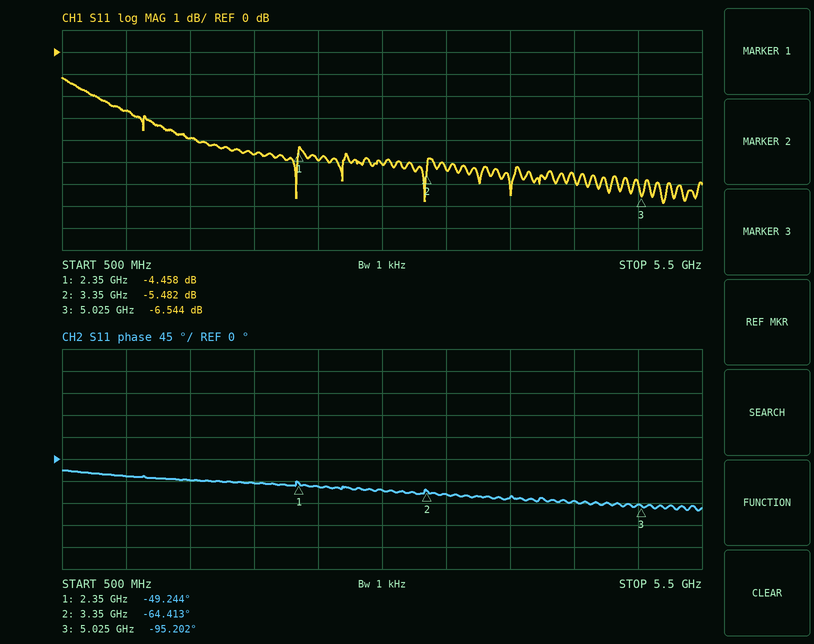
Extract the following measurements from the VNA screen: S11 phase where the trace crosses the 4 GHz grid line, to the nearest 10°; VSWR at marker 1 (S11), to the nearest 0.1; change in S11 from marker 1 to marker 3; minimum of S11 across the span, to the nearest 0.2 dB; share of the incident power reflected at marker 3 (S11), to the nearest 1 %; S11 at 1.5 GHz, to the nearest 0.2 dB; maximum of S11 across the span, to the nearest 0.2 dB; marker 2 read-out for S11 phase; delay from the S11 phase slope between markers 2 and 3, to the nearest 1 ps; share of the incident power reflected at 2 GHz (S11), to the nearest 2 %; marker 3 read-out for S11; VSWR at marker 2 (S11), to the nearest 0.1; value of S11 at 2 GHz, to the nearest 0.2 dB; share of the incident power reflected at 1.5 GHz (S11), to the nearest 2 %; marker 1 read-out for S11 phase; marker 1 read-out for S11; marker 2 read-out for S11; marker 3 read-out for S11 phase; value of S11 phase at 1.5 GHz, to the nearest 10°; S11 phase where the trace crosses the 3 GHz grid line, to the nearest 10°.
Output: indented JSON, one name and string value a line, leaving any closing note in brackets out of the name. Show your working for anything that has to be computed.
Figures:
{
  "S11 phase where the trace crosses the 4 GHz grid line, to the nearest 10°": "-80°",
  "VSWR at marker 1 (S11), to the nearest 0.1": "(1 + 0.5985)/(1 − 0.5985) ≈ 4.0",
  "change in S11 from marker 1 to marker 3": "-6.544 − (-4.458) = -2.086 dB",
  "minimum of S11 across the span, to the nearest 0.2 dB": "-6.8 dB",
  "share of the incident power reflected at marker 3 (S11), to the nearest 1 %": "10^(-6.544/10) ≈ 22 %",
  "S11 at 1.5 GHz, to the nearest 0.2 dB": "-4.0 dB",
  "maximum of S11 across the span, to the nearest 0.2 dB": "-1.2 dB",
  "marker 2 read-out for S11 phase": "-64.413°",
  "delay from the S11 phase slope between markers 2 and 3, to the nearest 1 ps": "−(-95.202° − (-64.413°))/(360° × 1.675 GHz) ≈ 51 ps",
  "share of the incident power reflected at 2 GHz (S11), to the nearest 2 %": "10^(-4.6/10) ≈ 34.7 %, so 34 % to the nearest 2 %",
  "marker 3 read-out for S11": "-6.544 dB",
  "VSWR at marker 2 (S11), to the nearest 0.1": "(1 + 0.5320)/(1 − 0.5320) ≈ 3.3",
  "value of S11 at 2 GHz, to the nearest 0.2 dB": "-4.6 dB",
  "share of the incident power reflected at 1.5 GHz (S11), to the nearest 2 %": "10^(-4/10) ≈ 40 %",
  "marker 1 read-out for S11 phase": "-49.244°",
  "marker 1 read-out for S11": "-4.458 dB",
  "marker 2 read-out for S11": "-5.482 dB",
  "marker 3 read-out for S11 phase": "-95.202°",
  "value of S11 phase at 1.5 GHz, to the nearest 10°": "-40°",
  "S11 phase where the trace crosses the 3 GHz grid line, to the nearest 10°": "-60°"
}
